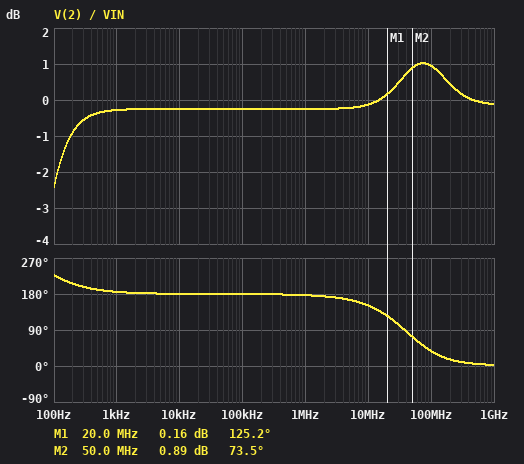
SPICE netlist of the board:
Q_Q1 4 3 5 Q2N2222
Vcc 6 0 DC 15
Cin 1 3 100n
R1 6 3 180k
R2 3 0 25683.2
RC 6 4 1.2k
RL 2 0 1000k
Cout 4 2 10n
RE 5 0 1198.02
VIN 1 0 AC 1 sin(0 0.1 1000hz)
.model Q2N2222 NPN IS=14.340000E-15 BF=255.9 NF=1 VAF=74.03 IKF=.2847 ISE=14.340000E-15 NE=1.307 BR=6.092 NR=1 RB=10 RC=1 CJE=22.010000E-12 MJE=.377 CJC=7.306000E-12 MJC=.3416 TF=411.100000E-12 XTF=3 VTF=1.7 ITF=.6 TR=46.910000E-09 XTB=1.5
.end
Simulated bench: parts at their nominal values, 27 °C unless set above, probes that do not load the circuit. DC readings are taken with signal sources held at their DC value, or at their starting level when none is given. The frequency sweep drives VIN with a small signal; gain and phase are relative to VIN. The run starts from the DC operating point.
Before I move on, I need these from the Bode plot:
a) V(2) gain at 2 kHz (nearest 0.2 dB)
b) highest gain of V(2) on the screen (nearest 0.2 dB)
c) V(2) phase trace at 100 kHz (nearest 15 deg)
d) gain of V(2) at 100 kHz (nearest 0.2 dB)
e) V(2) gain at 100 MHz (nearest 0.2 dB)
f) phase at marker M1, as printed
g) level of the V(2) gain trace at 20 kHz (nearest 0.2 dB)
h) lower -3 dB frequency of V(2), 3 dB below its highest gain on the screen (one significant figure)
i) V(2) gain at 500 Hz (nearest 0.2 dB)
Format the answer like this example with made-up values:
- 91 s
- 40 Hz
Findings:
- -0.2 dB
- 1.0 dB
- 180 deg
- -0.2 dB
- 1.0 dB
- 125.2 deg
- -0.2 dB
- 100 Hz
- -0.4 dB
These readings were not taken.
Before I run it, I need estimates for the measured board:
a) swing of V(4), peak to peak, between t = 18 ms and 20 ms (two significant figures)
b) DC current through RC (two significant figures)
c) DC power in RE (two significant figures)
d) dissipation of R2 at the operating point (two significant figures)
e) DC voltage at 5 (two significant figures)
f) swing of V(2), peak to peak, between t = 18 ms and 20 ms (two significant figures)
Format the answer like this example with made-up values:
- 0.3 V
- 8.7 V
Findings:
- 190 mV
- 920 µA
- 1.0 mW
- 120 µW
- 1.1 V
- 190 mV
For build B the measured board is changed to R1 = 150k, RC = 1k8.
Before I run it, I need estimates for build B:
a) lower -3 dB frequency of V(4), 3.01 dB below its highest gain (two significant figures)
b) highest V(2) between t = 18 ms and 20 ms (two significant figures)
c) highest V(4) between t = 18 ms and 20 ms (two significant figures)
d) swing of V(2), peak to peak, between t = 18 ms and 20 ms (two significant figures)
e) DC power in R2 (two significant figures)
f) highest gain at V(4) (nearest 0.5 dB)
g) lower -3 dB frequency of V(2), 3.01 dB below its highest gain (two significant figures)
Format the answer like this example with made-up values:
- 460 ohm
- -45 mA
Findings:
- 80 Hz
- 150 mV
- 13 V
- 290 mV
- 160 µW
- 3.5 dB
- 83 Hz
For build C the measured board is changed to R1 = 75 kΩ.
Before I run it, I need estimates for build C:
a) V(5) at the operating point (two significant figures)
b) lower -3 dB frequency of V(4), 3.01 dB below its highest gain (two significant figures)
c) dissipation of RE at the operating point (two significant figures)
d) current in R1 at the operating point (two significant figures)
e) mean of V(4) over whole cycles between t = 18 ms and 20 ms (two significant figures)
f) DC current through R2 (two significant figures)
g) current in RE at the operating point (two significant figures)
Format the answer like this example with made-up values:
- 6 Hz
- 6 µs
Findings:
- 2.9 V
- 120 Hz
- 7.0 mW
- 150 µA
- 12 V
- 140 µA
- 2.4 mA
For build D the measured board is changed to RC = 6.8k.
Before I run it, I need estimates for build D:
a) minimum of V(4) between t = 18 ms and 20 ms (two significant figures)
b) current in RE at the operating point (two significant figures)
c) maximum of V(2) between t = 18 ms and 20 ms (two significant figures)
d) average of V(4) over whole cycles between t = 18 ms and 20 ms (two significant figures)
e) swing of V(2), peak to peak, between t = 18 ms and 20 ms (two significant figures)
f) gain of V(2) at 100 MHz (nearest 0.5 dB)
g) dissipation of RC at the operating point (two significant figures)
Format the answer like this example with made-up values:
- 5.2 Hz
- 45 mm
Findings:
- 8.2 V
- 920 µA
- 540 mV
- 8.8 V
- 1.1 V
- 1.5 dB
- 5.7 mW
